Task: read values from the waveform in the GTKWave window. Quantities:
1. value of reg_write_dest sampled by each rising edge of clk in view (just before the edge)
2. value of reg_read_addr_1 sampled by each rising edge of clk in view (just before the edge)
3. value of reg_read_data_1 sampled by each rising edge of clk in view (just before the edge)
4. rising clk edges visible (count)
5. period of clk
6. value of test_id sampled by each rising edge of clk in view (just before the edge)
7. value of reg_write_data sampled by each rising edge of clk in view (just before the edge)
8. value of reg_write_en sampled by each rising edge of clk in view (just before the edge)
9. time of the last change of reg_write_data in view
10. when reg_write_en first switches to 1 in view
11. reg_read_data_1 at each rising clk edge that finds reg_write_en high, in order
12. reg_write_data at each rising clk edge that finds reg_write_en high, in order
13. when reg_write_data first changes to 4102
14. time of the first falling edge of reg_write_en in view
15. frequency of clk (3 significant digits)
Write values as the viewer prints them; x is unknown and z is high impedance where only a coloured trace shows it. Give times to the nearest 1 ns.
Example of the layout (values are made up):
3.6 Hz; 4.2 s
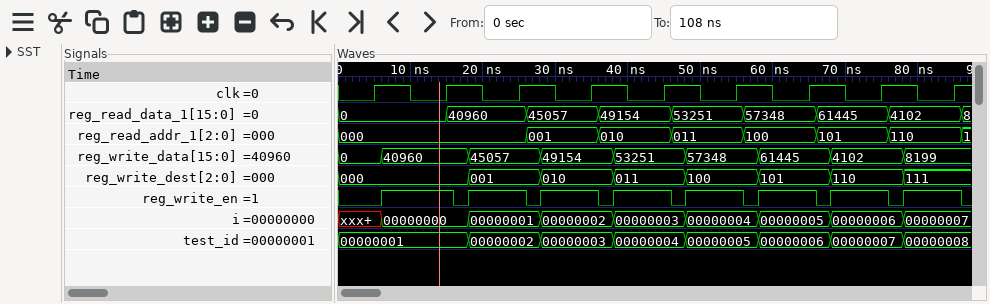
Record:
000, 000, 001, 010, 011, 100, 101, 110, 111; 000, 000, 000, 001, 010, 011, 100, 101, 110; 0, 0, 40960, 45057, 49154, 53251, 57348, 61445, 4102; 9; 10 ns; 00000001, 00000001, 00000002, 00000003, 00000004, 00000005, 00000006, 00000007, 00000008; 0, 40960, 45057, 49154, 53251, 57348, 61445, 4102, 8199; 0 1 1 1 1 1 1 1 1; 78 ns; 6 ns; 0, 40960, 45057, 49154, 53251, 57348, 61445, 4102; 40960, 45057, 49154, 53251, 57348, 61445, 4102, 8199; 68 ns; 16 ns; 100 MHz
